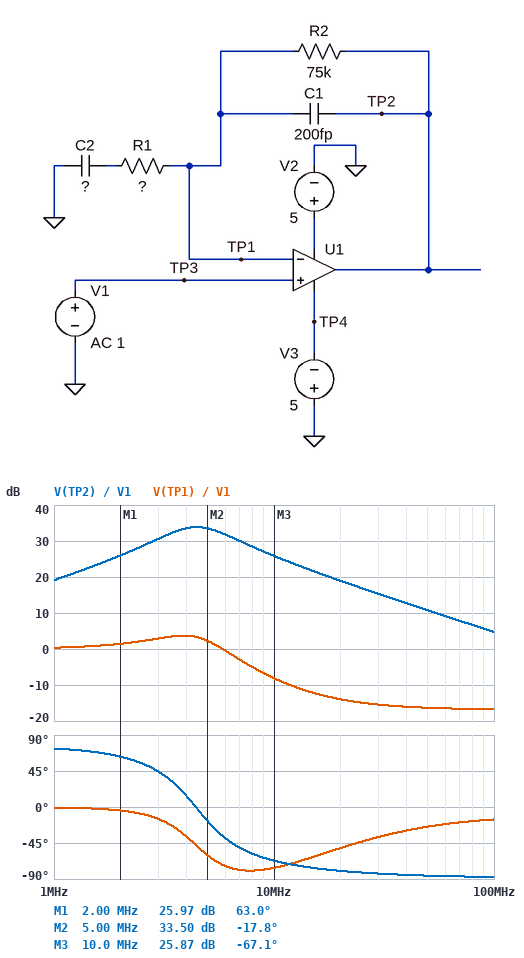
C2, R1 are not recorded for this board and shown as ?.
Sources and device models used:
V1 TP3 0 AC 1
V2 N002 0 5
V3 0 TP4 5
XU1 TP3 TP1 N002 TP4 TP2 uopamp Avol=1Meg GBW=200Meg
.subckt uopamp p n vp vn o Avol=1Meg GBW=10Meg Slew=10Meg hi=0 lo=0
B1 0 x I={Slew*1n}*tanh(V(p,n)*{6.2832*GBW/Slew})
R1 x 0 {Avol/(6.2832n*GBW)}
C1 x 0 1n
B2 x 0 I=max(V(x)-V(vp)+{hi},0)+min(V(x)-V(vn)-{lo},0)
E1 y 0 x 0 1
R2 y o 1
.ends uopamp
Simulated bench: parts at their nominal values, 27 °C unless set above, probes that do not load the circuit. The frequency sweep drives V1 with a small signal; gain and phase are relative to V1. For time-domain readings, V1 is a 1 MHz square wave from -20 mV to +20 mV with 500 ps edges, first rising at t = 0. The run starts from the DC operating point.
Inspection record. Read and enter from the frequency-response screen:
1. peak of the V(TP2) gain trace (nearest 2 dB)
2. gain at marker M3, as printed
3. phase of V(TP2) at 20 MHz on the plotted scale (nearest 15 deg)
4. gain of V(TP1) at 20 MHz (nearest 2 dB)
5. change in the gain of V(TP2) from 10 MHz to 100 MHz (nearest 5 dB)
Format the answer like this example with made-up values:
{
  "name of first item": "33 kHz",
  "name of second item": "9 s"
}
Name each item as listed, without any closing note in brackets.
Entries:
{
  "peak of the V(TP2) gain trace": "34 dB",
  "gain at marker M3, as printed": "25.87 dB",
  "phase of V(TP2) at 20 MHz on the plotted scale": "-75 deg",
  "gain of V(TP1) at 20 MHz": "-14 dB",
  "change in the gain of V(TP2) from 10 MHz to 100 MHz": "-20 dB"
}
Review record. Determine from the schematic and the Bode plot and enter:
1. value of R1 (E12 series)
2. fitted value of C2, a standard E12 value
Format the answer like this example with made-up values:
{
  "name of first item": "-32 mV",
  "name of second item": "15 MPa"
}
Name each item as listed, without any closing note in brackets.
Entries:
{
  "value of R1": "680 Ω",
  "fitted value of C2, a standard E12 value": "18 pF"
}
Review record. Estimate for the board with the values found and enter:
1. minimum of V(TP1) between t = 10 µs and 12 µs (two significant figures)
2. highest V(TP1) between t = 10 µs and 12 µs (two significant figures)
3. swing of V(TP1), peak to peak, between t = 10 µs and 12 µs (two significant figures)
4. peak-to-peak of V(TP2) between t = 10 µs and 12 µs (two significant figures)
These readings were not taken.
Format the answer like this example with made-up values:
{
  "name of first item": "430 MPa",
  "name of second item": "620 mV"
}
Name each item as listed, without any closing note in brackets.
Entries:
{
  "minimum of V(TP1) between t = 10 µs and 12 µs": "-33 mV",
  "highest V(TP1) between t = 10 µs and 12 µs": "33 mV",
  "swing of V(TP1), peak to peak, between t = 10 µs and 12 µs": "66 mV",
  "peak-to-peak of V(TP2) between t = 10 µs and 12 µs": "1.5 V"
}
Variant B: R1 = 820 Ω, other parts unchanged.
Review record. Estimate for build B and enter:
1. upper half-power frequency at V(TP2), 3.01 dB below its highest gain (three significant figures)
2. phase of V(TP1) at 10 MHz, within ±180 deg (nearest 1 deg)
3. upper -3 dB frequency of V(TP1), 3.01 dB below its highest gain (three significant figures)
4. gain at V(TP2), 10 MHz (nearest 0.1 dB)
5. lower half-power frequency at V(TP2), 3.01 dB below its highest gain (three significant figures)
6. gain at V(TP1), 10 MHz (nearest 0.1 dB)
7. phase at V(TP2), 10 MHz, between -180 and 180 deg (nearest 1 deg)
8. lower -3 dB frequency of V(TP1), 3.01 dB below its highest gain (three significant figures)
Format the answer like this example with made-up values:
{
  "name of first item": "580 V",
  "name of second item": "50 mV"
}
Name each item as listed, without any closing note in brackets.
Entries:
{
  "upper half-power frequency at V(TP2), 3.01 dB below its highest gain": "6.60 MHz",
  "phase of V(TP1) at 10 MHz, within ±180 deg": "-70 deg",
  "upper -3 dB frequency of V(TP1), 3.01 dB below its highest gain": "5.57 MHz",
  "gain at V(TP2), 10 MHz": "25.5 dB",
  "lower half-power frequency at V(TP2), 3.01 dB below its highest gain": "2.92 MHz",
  "gain at V(TP1), 10 MHz": "-7.8 dB",
  "phase at V(TP2), 10 MHz, between -180 and 180 deg": "-66 deg",
  "lower -3 dB frequency of V(TP1), 3.01 dB below its highest gain": "925 kHz"
}
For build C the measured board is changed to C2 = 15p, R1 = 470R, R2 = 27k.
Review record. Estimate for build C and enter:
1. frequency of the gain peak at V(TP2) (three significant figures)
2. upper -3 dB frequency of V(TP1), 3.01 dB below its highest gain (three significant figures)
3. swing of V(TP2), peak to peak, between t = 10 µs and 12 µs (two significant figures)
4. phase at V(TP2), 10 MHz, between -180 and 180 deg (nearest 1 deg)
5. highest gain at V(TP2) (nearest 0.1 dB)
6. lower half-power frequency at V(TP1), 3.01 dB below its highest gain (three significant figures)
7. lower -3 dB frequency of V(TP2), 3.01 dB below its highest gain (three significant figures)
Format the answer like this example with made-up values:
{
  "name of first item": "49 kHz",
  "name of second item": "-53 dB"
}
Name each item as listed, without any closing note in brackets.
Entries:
{
  "frequency of the gain peak at V(TP2)": "8.28 MHz",
  "upper -3 dB frequency of V(TP1), 3.01 dB below its highest gain": "10.1 MHz",
  "swing of V(TP2), peak to peak, between t = 10 µs and 12 µs": "840 mV",
  "phase at V(TP2), 10 MHz, between -180 and 180 deg": "-31 deg",
  "highest gain at V(TP2)": "30.0 dB",
  "lower half-power frequency at V(TP1), 3.01 dB below its highest gain": "3.69 MHz",
  "lower -3 dB frequency of V(TP2), 3.01 dB below its highest gain": "5.91 MHz"
}
